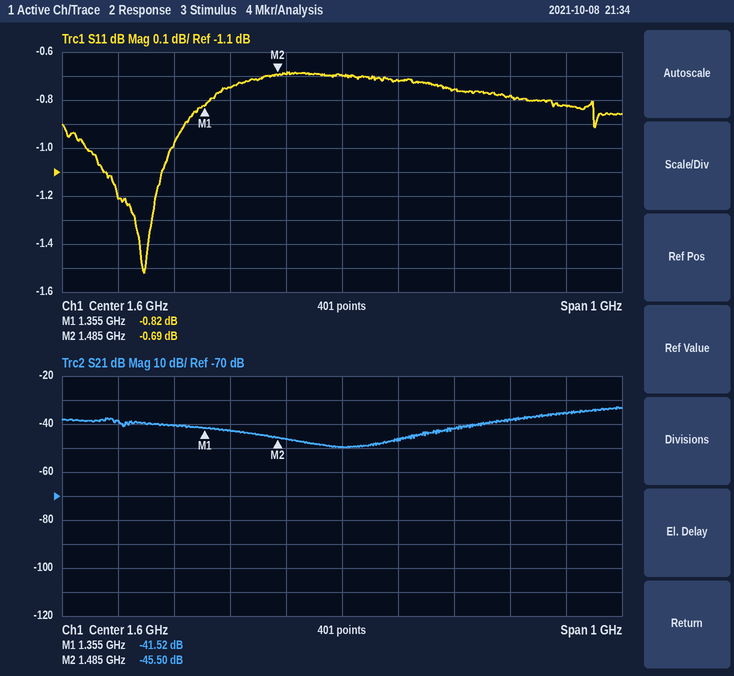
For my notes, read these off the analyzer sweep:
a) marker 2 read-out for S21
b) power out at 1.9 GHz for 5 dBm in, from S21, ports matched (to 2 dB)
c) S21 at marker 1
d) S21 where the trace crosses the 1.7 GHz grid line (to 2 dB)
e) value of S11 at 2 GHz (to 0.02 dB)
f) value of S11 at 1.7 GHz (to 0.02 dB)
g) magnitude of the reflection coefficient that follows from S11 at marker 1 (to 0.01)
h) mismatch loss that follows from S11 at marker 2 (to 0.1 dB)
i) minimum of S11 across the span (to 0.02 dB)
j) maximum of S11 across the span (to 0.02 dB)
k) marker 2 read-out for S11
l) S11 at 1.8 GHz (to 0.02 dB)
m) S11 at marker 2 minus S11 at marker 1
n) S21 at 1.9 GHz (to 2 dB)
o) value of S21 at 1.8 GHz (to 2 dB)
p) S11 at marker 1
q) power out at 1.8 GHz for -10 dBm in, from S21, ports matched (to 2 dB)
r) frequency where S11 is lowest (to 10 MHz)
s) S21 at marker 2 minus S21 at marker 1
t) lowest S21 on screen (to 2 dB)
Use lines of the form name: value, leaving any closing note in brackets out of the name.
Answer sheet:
marker 2 read-out for S21: -45.50 dB
power out at 1.9 GHz for 5 dBm in, from S21, ports matched: -34 dBm
S21 at marker 1: -41.52 dB
S21 where the trace crosses the 1.7 GHz grid line: -46 dB
value of S11 at 2 GHz: -0.82 dB
value of S11 at 1.7 GHz: -0.72 dB
magnitude of the reflection coefficient that follows from S11 at marker 1: 0.91
mismatch loss that follows from S11 at marker 2: 8.3 dB
minimum of S11 across the span: -1.52 dB
maximum of S11 across the span: -0.68 dB
marker 2 read-out for S11: -0.69 dB
S11 at 1.8 GHz: -0.76 dB
S11 at marker 2 minus S11 at marker 1: 0.13 dB
S21 at 1.9 GHz: -38 dB
value of S21 at 1.8 GHz: -42 dB
S11 at marker 1: -0.82 dB
power out at 1.8 GHz for -10 dBm in, from S21, ports matched: -52 dBm
frequency where S11 is lowest: 1.25 GHz
S21 at marker 2 minus S21 at marker 1: -3.98 dB
lowest S21 on screen: -50 dB
